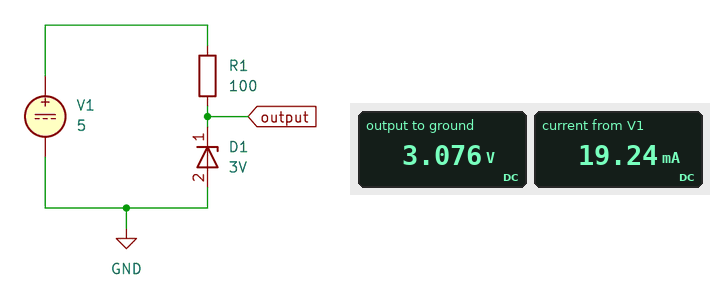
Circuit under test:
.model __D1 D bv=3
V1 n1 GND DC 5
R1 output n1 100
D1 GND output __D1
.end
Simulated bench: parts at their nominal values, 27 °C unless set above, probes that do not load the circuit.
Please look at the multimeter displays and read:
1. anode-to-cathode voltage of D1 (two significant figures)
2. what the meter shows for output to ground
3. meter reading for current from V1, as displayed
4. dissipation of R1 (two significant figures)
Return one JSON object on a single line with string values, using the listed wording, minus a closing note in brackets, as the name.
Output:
{"anode-to-cathode voltage of D1": "-3.1 V", "what the meter shows for output to ground": "3.076 V", "meter reading for current from V1, as displayed": "19.24 mA", "dissipation of R1": "37 mW"}
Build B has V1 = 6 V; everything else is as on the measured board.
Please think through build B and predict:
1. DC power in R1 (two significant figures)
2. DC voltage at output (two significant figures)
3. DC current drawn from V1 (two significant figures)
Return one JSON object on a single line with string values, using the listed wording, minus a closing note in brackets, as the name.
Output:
{"DC power in R1": "85 mW", "DC voltage at output": "3.1 V", "DC current drawn from V1": "29 mA"}
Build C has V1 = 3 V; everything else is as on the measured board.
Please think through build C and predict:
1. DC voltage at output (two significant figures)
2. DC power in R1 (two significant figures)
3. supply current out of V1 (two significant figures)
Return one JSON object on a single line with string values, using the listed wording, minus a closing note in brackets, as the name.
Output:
{"DC voltage at output": "3.0 V", "DC power in R1": "9.4 µW", "supply current out of V1": "310 µA"}
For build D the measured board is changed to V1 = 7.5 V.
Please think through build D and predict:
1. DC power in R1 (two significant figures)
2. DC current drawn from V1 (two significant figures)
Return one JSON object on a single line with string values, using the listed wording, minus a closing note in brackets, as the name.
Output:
{"DC power in R1": "190 mW", "DC current drawn from V1": "44 mA"}
